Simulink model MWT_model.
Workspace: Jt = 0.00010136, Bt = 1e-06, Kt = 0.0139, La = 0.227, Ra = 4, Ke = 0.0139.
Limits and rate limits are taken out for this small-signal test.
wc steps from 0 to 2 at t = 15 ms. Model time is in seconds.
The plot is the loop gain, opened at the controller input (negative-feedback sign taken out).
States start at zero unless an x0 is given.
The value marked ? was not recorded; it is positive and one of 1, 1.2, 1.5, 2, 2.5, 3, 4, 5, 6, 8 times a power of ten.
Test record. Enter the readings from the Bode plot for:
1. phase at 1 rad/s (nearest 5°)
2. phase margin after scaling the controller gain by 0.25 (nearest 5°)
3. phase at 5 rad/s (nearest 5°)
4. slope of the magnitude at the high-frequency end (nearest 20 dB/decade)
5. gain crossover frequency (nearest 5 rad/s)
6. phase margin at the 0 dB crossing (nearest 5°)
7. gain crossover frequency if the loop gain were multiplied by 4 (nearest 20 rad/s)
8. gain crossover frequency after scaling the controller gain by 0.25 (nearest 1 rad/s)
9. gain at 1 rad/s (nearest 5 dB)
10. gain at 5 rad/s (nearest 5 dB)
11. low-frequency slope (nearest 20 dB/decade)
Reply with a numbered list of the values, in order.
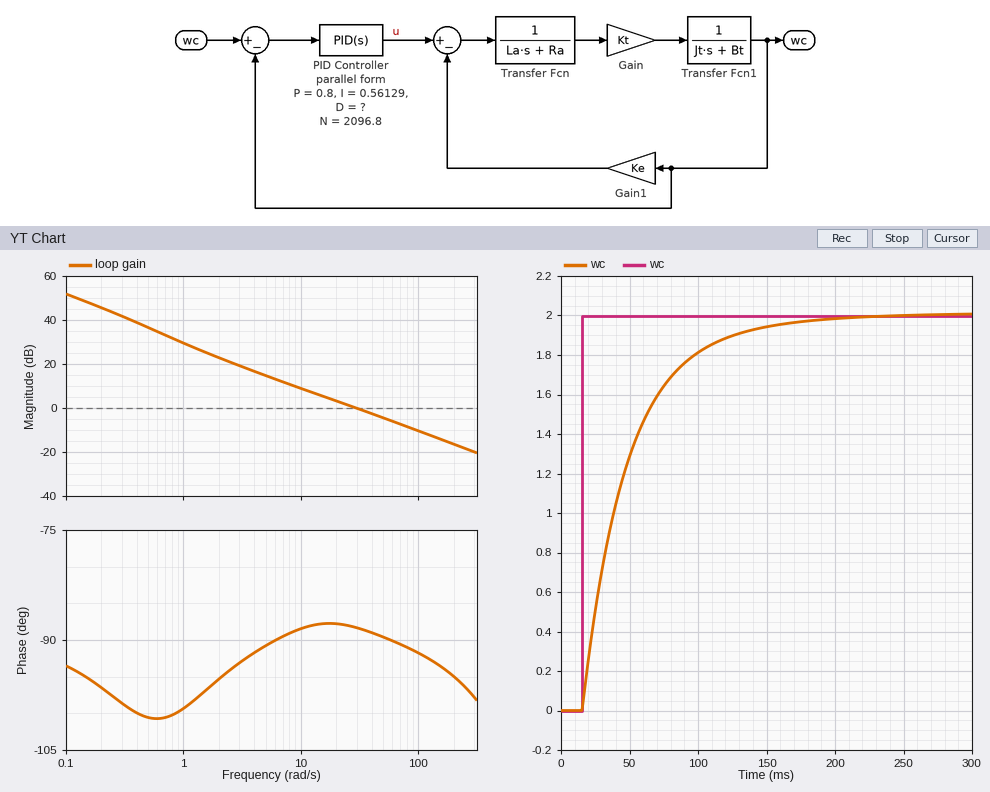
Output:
1. -100°
2. 90°
3. -90°
4. -20 dB/decade
5. 30 rad/s
6. 90°
7. 120 rad/s
8. 7 rad/s
9. 30 dB
10. 15 dB
11. -20 dB/decade
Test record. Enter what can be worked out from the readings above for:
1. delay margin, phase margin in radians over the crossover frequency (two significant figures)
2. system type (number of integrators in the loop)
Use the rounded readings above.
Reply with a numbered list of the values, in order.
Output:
1. 0.052 s
2. 1
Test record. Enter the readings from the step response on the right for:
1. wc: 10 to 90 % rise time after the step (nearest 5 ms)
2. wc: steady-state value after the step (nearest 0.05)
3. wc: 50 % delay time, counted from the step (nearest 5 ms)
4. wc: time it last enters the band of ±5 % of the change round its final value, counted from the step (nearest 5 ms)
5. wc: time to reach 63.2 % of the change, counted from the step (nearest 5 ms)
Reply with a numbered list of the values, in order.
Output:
1. 80 ms
2. 2.00
3. 25 ms
4. 115 ms
5. 35 ms
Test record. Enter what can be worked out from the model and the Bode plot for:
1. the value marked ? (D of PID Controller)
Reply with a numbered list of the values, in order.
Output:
1. 0.05
